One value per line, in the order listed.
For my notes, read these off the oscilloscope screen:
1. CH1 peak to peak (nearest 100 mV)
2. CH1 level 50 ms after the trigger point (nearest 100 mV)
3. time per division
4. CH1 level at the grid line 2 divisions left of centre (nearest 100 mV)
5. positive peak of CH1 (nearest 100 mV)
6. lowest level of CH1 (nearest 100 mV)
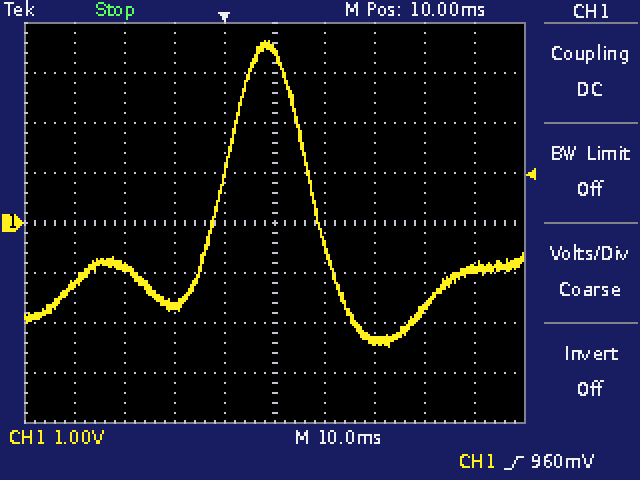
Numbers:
6.1 V
-900 mV
10 ms
-1.7 V
3.6 V
-2.5 V
